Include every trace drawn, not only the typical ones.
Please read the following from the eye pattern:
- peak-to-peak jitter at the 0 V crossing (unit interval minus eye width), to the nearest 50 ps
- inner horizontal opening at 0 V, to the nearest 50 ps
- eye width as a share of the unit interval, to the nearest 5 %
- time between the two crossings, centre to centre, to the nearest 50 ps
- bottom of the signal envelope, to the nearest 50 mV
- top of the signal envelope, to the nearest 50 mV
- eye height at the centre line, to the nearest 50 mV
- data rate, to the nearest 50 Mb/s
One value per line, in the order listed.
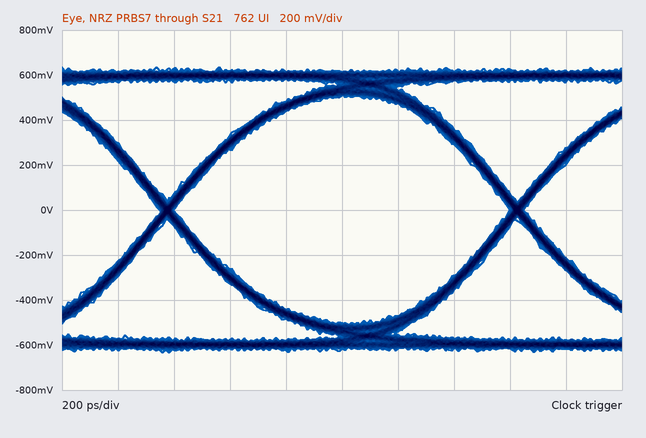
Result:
50 ps
1.20 ns
95 %
1.25 ns
-650 mV
650 mV
1.00 V
800 Mb/s
